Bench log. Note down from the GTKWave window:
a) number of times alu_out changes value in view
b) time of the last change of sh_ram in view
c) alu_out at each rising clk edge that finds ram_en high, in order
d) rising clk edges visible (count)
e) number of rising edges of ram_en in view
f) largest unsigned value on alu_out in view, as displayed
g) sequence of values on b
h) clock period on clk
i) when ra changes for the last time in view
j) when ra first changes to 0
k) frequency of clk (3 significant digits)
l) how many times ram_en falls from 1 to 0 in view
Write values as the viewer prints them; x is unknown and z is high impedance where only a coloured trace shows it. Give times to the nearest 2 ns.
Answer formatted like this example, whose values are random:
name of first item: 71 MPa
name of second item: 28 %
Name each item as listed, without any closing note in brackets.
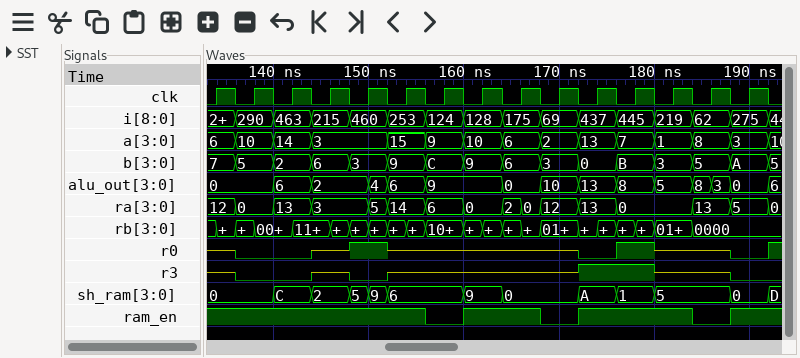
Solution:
number of times alu_out changes value in view: 14
time of the last change of sh_ram in view: 192 ns
alu_out at each rising clk edge that finds ram_en high, in order: 0, 0, 6, 2, 2, 6, 9, 0, 13, 8, 5, 0
rising clk edges visible: 15
number of rising edges of ram_en in view: 3
largest unsigned value on alu_out in view, as displayed: 13
sequence of values on b: 7, 5, 2, 6, 3, 9, C, 9, 6, 3, 0, B, 3, 5, A, 5
clock period on clk: 4 ns
when ra changes for the last time in view: 192 ns
when ra first changes to 0: 136 ns
frequency of clk: 250 MHz
how many times ram_en falls from 1 to 0 in view: 3
